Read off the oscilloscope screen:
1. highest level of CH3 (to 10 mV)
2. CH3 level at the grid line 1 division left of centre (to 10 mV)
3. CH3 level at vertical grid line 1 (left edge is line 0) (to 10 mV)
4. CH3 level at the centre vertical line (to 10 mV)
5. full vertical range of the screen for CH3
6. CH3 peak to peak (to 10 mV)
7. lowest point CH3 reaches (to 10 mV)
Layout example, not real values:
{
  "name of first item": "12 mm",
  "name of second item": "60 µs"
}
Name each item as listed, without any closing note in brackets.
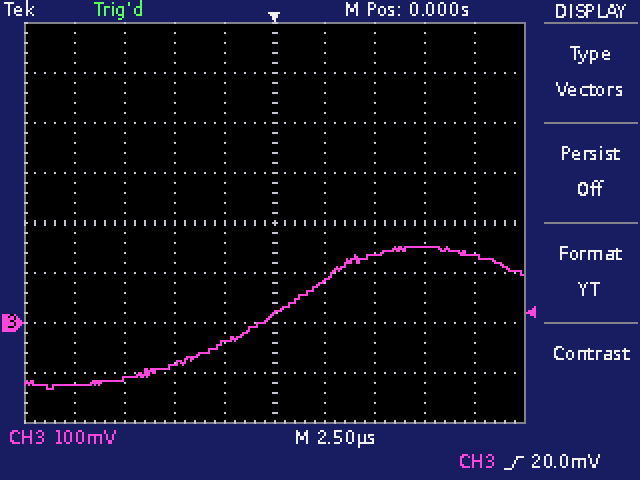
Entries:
{
  "highest level of CH3": "150 mV",
  "CH3 level at the grid line 1 division left of centre": "-40 mV",
  "CH3 level at vertical grid line 1 (left edge is line 0)": "-120 mV",
  "CH3 level at the centre vertical line": "20 mV",
  "full vertical range of the screen for CH3": "800 mV",
  "CH3 peak to peak": "280 mV",
  "lowest point CH3 reaches": "-130 mV"
}
